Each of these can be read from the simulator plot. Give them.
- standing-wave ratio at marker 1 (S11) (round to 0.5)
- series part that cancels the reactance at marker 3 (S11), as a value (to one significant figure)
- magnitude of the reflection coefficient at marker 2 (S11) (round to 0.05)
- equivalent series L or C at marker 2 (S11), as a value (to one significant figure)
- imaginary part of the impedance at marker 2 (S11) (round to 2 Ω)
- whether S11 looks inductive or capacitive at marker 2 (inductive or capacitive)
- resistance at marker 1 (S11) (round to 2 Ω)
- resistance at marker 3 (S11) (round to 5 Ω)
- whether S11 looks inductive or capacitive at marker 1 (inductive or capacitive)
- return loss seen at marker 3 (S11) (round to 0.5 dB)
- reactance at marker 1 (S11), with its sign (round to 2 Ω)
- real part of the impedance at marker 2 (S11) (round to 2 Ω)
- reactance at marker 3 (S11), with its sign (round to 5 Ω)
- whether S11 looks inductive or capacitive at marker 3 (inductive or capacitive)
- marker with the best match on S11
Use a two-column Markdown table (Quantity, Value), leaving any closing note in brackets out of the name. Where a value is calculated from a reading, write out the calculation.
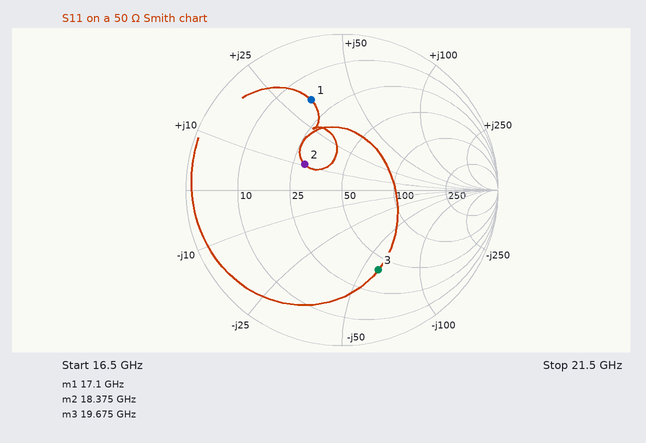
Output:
| Quantity | Value |
|---|---|
| standing-wave ratio at marker 1 (S11) | 4.0 |
| series part that cancels the reactance at marker 3 (S11), as a value | L = 60 Ω/(2π × 19.675 GHz) ≈ 485 pH, so 500 pH to one significant figure |
| magnitude of the reflection coefficient at marker 2 (S11) | 0.30 |
| equivalent series L or C at marker 2 (S11), as a value | L = 10 Ω/(2π × 18.375 GHz) ≈ 86.6 pH, so 90 pH to one significant figure |
| imaginary part of the impedance at marker 2 (S11) | +10 Ω |
| whether S11 looks inductive or capacitive at marker 2 | inductive |
| resistance at marker 1 (S11) | 18 Ω |
| resistance at marker 3 (S11) | 40 Ω |
| whether S11 looks inductive or capacitive at marker 1 | inductive |
| return loss seen at marker 3 (S11) | 5.0 dB |
| reactance at marker 1 (S11), with its sign | +32 Ω |
| real part of the impedance at marker 2 (S11) | 30 Ω |
| reactance at marker 3 (S11), with its sign | -60 Ω |
| whether S11 looks inductive or capacitive at marker 3 | capacitive |
| marker with the best match on S11 | marker 2 |
